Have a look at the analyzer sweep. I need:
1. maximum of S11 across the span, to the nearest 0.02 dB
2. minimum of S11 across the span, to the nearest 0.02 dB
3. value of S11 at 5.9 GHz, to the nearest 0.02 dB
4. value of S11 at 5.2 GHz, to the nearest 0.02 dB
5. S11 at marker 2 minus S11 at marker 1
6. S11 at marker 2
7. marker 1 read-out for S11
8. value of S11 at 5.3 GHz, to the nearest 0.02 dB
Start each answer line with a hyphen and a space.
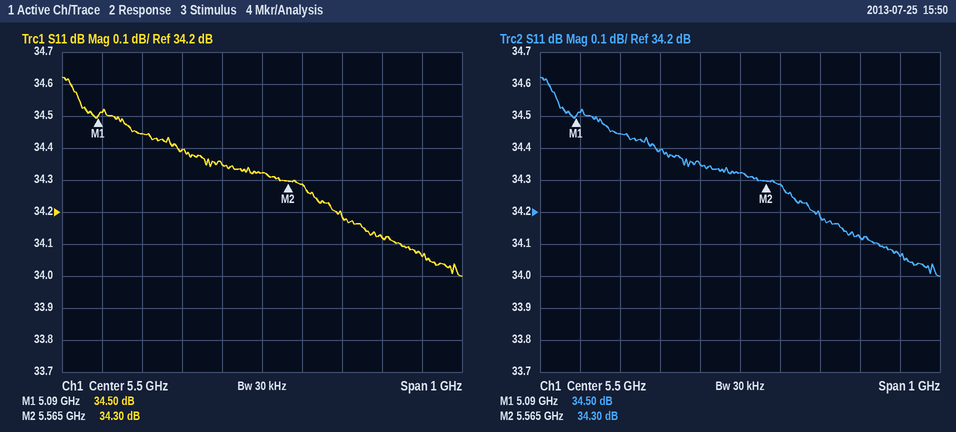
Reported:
- 34.62 dB
- 34.00 dB
- 34.06 dB
- 34.44 dB
- -0.20 dB
- 34.30 dB
- 34.50 dB
- 34.40 dB
